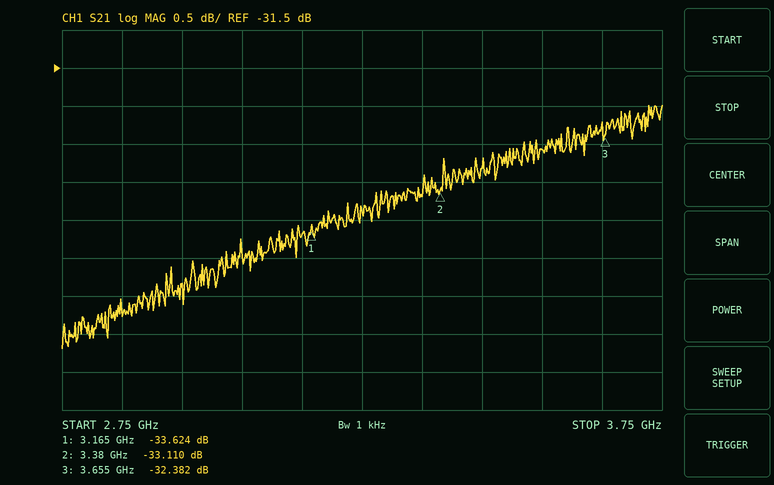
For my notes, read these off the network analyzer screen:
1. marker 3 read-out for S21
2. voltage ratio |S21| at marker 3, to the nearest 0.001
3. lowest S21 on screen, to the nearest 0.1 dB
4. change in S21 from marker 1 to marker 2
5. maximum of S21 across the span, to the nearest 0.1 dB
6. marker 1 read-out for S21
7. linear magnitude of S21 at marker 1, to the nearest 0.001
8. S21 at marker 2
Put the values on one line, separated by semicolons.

-32.382 dB; 0.024; -35.2 dB; 0.514 dB; -32.0 dB; -33.624 dB; 0.021; -33.110 dB
